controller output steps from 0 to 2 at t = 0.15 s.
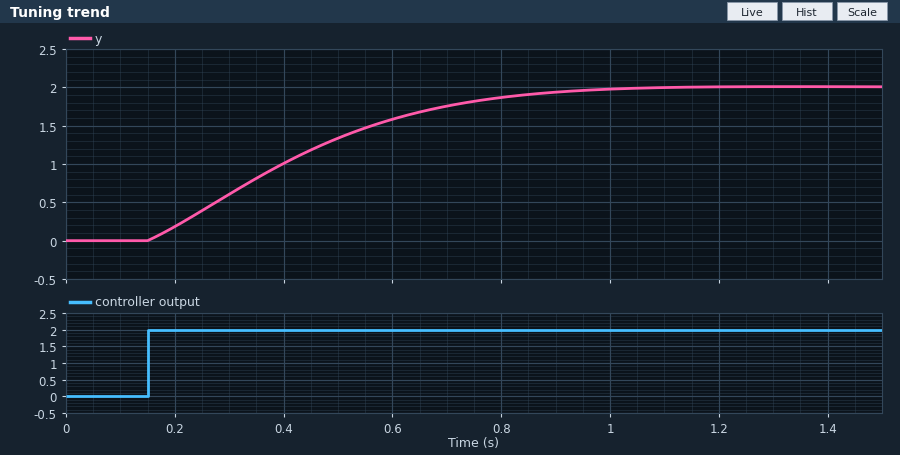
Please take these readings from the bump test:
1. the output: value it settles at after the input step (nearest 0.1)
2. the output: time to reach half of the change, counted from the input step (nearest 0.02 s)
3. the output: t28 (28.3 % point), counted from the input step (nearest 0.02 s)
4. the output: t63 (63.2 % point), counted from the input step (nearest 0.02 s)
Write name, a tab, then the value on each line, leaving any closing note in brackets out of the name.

the output: value it settles at after the input step	2.0
the output: time to reach half of the change, counted from the input step	0.24 s
the output: t28 (28.3 % point), counted from the input step	0.14 s
the output: t63 (63.2 % point), counted from the input step	0.32 s
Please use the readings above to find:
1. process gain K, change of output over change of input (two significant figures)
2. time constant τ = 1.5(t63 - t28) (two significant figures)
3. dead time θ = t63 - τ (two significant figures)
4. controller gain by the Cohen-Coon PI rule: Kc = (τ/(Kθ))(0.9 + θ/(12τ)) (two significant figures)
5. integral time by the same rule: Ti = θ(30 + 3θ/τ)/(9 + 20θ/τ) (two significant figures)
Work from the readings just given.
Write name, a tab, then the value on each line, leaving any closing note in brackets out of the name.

process gain K, change of output over change of input	1.0
time constant τ = 1.5(t63 - t28)	0.27 s
dead time θ = t63 - τ	0.050 s
controller gain by the Cohen-Coon PI rule: Kc = (τ/(Kθ))(0.9 + θ/(12τ))	4.9
integral time by the same rule: Ti = θ(30 + 3θ/τ)/(9 + 20θ/τ)	0.12 s
